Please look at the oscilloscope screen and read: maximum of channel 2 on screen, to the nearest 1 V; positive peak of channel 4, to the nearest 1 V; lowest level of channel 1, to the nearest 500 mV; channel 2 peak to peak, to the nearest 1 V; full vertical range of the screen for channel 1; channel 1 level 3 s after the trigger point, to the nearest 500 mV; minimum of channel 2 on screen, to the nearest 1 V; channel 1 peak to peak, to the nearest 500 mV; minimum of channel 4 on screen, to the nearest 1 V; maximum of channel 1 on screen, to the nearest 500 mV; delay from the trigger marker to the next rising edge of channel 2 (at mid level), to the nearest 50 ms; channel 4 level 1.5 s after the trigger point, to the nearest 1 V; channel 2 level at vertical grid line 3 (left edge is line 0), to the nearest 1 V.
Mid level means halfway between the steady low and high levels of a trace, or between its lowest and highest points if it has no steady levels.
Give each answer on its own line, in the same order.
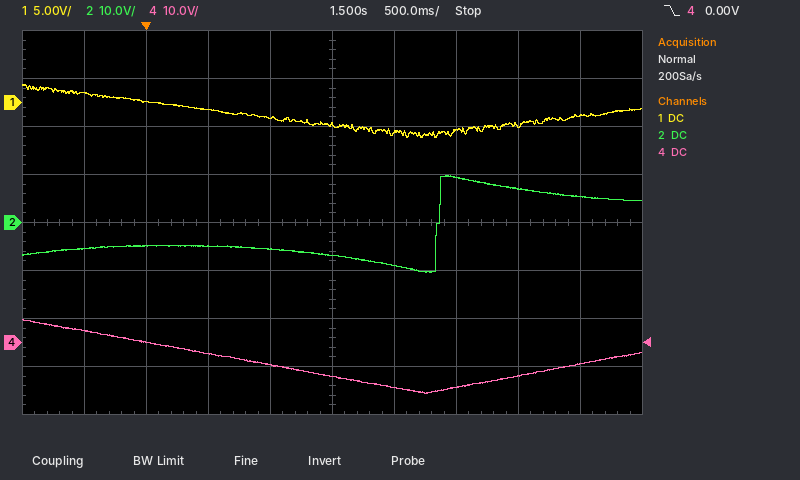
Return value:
10 V
5 V
-3.5 V
20 V
40 V
-2.5 V
-10 V
5.5 V
-11 V
2.0 V
2.35 s
-7 V
-5 V
